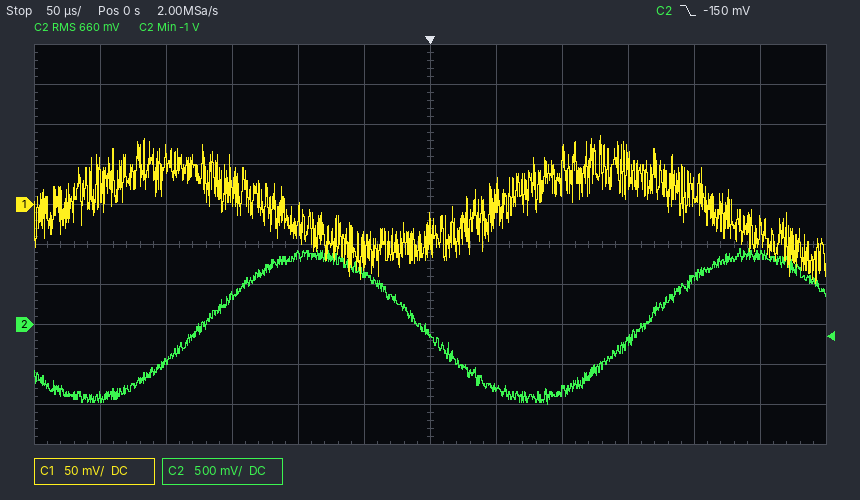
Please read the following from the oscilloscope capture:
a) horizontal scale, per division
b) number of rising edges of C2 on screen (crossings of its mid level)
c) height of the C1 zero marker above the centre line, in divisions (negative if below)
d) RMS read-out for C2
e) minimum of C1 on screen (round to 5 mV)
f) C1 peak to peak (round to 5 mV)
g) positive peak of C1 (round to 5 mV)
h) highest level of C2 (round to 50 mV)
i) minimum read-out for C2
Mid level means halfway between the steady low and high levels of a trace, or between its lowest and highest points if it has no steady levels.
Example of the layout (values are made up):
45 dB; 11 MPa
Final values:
50 µs; 2; +1.0 div; 660 mV; -100 mV; 185 mV; 85 mV; 950 mV; -1 V
